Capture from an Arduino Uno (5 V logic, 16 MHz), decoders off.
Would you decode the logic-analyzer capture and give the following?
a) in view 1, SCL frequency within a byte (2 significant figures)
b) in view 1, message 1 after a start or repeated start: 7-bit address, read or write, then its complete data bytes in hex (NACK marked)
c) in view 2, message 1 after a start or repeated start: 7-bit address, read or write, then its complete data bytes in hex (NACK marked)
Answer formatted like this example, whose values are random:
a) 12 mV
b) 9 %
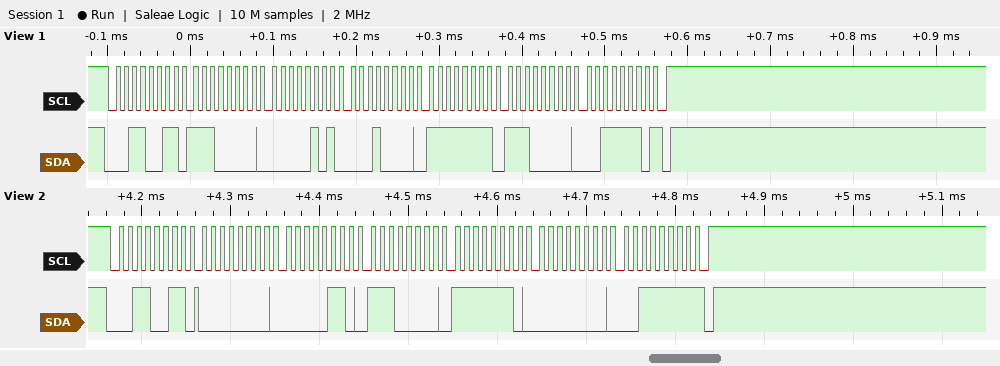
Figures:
a) 100 kHz
b) 0x19 read: E0 05 10 FF E0 3E NACK
c) 0x19 read: 00 06 E0 FE 00 3F NACK
